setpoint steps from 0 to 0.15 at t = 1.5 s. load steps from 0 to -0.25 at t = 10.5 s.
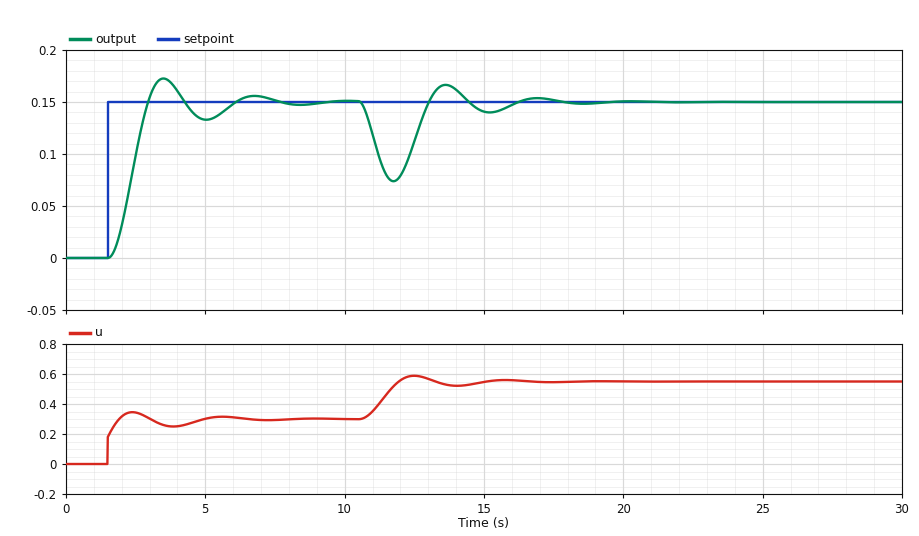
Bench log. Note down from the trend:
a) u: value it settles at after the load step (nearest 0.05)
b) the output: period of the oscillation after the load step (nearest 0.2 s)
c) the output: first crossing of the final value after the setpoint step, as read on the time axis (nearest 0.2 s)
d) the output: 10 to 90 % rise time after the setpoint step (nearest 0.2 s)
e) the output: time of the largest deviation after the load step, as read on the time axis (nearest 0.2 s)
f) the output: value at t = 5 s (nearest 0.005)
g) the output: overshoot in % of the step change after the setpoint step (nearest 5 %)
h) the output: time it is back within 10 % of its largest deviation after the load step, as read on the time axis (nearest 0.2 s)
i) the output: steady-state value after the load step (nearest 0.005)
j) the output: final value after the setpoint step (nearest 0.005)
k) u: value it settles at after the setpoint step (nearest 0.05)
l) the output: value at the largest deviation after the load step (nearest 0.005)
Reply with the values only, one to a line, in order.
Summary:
0.55
3.4 s
3.0 s
1.0 s
11.8 s
0.135
15 %
15.6 s
0.150
0.150
0.30
0.075
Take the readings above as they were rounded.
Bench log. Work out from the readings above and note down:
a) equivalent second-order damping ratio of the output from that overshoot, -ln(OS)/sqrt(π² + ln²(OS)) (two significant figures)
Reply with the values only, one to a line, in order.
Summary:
0.52
